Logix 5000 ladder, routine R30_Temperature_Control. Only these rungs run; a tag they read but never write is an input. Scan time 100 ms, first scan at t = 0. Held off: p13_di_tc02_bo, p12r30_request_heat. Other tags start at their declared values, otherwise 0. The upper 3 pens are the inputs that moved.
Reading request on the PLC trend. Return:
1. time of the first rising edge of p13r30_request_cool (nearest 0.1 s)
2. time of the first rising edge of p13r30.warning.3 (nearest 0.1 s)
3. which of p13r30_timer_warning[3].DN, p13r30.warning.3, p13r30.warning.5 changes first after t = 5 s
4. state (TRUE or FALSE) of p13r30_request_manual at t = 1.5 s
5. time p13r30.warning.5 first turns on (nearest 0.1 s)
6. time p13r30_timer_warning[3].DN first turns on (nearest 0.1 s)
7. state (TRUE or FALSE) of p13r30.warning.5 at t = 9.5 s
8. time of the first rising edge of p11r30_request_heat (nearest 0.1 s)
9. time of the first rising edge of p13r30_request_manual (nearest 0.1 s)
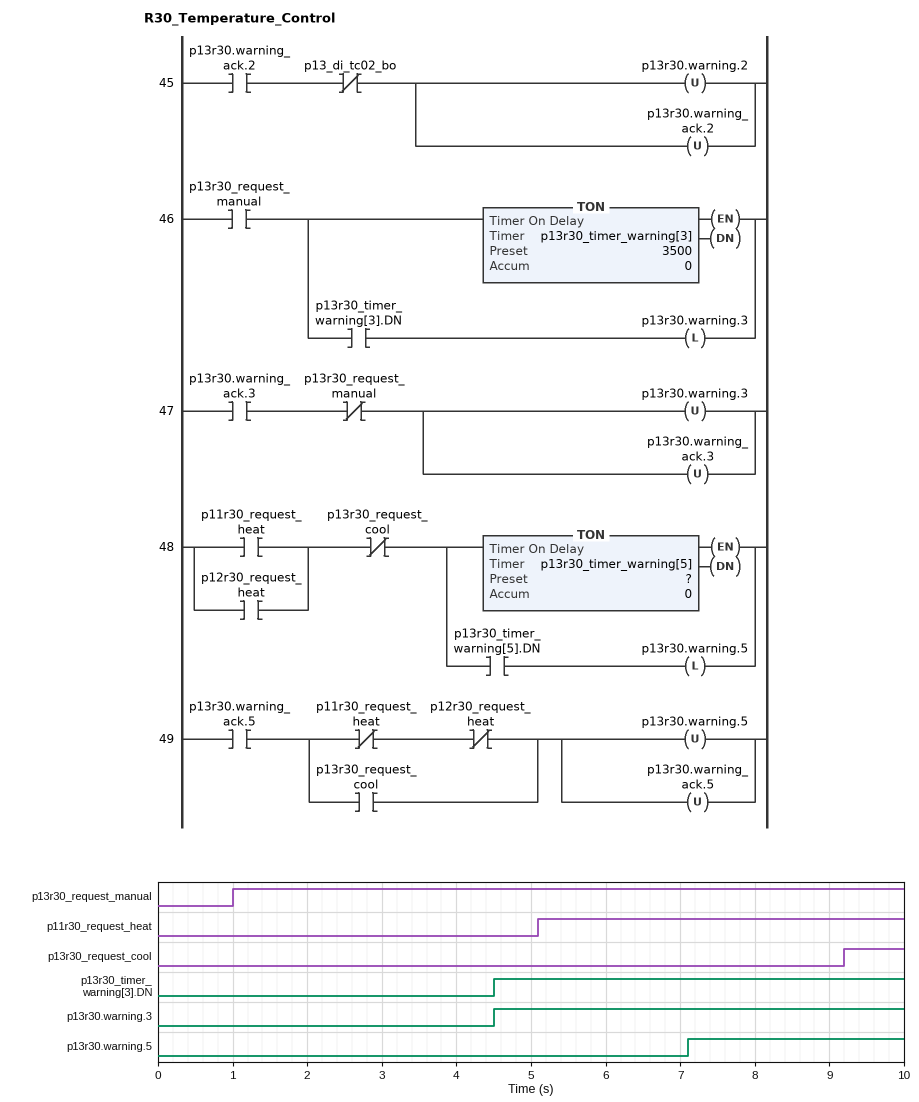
9.2 s
4.5 s
p13r30.warning.5
TRUE
7.1 s
4.5 s
TRUE
5.1 s
1.0 s
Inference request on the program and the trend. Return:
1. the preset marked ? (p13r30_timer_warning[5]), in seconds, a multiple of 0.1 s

2.0 s
